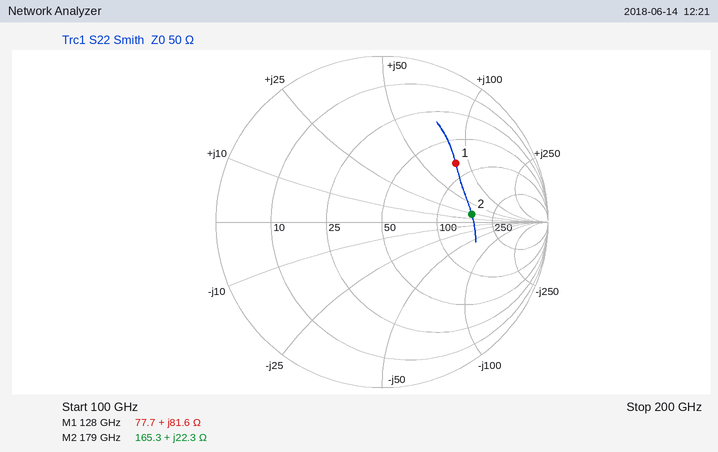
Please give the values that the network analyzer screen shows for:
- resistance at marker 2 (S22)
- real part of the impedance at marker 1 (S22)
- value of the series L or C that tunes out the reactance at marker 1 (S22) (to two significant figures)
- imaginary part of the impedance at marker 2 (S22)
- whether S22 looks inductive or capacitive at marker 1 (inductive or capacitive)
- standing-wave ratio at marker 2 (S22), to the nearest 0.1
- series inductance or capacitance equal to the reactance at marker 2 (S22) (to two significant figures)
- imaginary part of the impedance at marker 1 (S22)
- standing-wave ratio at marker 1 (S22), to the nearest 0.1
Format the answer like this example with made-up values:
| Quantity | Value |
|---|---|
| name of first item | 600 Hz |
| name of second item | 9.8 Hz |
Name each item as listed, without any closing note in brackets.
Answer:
| Quantity | Value |
|---|---|
| resistance at marker 2 | 165.3 Ω |
| real part of the impedance at marker 1 | 77.7 Ω |
| value of the series L or C that tunes out the reactance at marker 1 (S22) | 15 fF |
| imaginary part of the impedance at marker 2 | +22.3 Ω |
| whether S22 looks inductive or capacitive at marker 1 | inductive |
| standing-wave ratio at marker 2 (S22), to the nearest 0.1 | 3.4 |
| series inductance or capacitance equal to the reactance at marker 2 (S22) | 20 pH |
| imaginary part of the impedance at marker 1 | +81.6 Ω |
| standing-wave ratio at marker 1 (S22), to the nearest 0.1 | 3.6 |
